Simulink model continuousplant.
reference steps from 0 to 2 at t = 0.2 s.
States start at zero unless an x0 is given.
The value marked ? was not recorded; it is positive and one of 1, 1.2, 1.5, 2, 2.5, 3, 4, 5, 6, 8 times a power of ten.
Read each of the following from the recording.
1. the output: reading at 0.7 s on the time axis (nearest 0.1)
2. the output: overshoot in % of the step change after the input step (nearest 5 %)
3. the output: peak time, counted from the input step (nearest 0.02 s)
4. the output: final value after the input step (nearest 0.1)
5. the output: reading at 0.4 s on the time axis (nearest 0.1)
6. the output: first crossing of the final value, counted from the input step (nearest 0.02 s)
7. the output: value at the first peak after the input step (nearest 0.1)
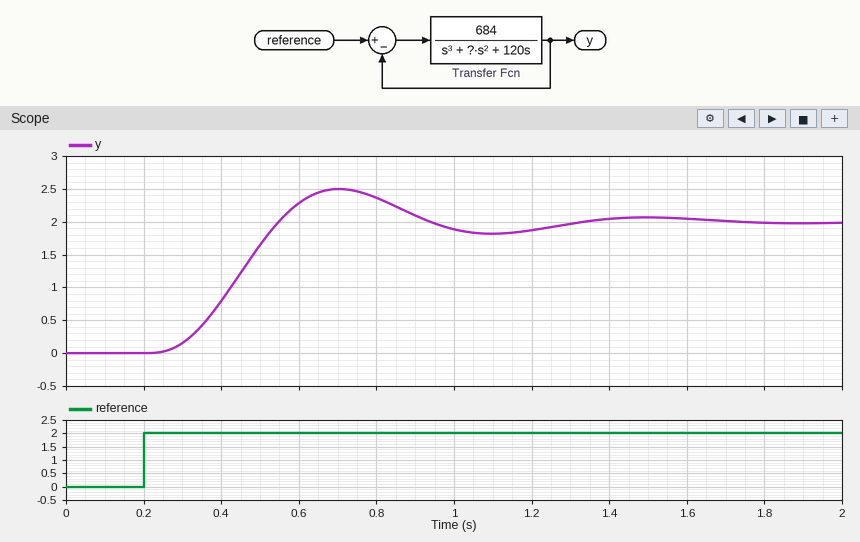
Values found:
2.5
25 %
0.50 s
2.0
0.8
0.34 s
2.5
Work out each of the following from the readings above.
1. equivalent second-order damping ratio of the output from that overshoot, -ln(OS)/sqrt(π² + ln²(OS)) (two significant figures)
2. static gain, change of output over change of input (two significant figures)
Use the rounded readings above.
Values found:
0.40
1.0
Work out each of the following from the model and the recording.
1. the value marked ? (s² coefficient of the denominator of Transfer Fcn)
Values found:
15
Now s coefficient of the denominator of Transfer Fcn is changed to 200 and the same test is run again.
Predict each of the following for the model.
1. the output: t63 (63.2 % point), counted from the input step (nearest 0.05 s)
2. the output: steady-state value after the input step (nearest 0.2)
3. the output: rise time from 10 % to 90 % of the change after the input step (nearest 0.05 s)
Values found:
0.30 s
2.0
0.40 s
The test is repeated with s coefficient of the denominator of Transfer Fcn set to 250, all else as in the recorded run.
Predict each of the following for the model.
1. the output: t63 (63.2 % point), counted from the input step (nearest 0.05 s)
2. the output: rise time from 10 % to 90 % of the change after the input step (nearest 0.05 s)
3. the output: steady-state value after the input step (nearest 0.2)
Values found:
0.35 s
0.65 s
2.0
